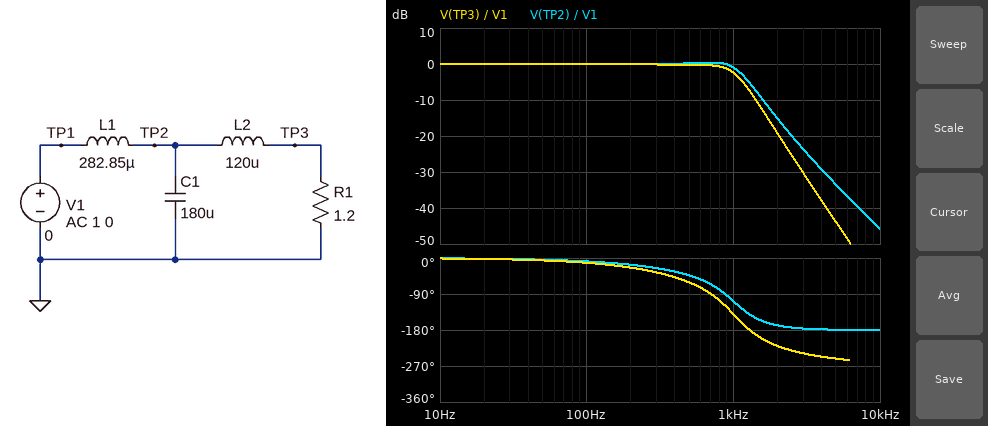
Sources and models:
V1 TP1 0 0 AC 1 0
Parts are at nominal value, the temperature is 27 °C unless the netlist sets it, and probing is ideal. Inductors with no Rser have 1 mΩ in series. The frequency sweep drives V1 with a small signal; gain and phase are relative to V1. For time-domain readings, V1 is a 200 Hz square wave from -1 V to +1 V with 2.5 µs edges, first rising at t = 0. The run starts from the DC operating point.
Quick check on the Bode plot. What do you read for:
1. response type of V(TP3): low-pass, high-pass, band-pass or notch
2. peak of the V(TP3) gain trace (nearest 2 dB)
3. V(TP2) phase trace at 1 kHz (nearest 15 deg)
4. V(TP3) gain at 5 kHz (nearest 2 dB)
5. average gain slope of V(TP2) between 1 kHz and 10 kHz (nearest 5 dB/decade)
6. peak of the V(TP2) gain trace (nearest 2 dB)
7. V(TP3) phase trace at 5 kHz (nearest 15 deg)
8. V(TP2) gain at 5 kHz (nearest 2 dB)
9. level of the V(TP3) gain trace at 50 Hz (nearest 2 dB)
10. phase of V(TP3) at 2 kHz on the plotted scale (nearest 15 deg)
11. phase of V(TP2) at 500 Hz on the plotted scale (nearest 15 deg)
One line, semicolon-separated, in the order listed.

low-pass; 0 dB; -105 deg; -44 dB; -45 dB/decade; 0 dB; -255 deg; -34 dB; 0 dB; -225 deg; -45 deg
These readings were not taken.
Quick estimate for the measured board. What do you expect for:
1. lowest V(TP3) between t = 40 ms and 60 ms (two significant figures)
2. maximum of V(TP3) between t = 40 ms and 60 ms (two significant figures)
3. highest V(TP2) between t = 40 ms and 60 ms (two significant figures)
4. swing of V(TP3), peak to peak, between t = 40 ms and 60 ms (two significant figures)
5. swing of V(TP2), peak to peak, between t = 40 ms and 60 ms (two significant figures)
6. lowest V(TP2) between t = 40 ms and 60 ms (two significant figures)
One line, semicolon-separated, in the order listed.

-1.2 V; 1.2 V; 1.2 V; 2.3 V; 2.5 V; -1.2 V
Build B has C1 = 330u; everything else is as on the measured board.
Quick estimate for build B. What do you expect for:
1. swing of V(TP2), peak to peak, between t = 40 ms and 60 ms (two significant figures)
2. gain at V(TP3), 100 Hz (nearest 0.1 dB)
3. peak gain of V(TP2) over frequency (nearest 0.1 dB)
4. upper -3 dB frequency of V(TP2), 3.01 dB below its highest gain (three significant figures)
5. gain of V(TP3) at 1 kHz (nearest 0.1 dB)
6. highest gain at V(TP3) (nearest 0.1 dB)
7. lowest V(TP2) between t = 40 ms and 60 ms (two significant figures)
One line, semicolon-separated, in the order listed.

3.0 V; 0.1 dB; 2.7 dB; 725 Hz; -8.6 dB; 2.3 dB; -1.5 V
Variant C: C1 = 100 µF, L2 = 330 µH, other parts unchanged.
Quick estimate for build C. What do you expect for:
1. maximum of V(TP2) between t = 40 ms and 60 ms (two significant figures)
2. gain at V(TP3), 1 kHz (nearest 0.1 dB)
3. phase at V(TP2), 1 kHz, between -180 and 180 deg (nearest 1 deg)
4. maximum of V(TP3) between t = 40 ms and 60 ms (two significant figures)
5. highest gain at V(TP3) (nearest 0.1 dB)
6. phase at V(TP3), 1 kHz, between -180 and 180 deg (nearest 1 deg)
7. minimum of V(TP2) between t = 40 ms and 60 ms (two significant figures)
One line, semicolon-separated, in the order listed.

1.4 V; -2.2 dB; -35 deg; 1.1 V; 2.2 dB; -95 deg; -1.4 V
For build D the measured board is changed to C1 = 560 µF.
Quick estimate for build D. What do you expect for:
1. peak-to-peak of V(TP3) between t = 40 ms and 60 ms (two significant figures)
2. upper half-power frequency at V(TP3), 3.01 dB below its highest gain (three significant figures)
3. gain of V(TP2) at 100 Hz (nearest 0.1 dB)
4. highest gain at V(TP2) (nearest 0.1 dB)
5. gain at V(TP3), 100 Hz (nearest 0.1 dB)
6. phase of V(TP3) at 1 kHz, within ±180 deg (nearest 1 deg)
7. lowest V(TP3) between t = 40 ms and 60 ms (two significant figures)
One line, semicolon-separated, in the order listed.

3.2 V; 510 Hz; 0.4 dB; 4.8 dB; 0.3 dB; 161 deg; -1.6 V
